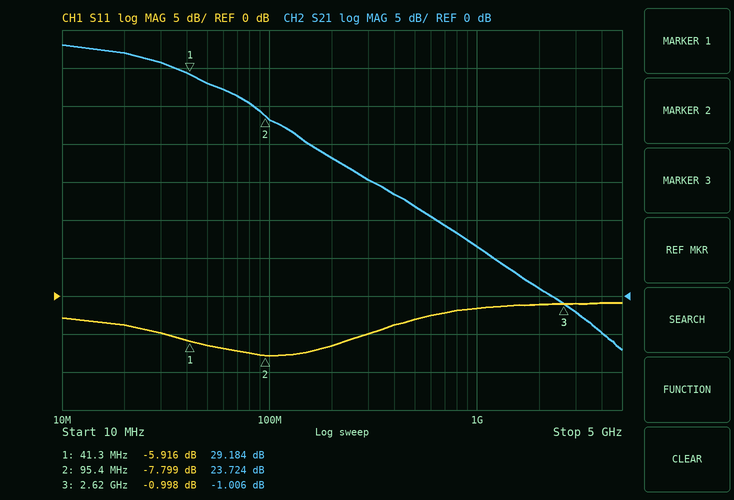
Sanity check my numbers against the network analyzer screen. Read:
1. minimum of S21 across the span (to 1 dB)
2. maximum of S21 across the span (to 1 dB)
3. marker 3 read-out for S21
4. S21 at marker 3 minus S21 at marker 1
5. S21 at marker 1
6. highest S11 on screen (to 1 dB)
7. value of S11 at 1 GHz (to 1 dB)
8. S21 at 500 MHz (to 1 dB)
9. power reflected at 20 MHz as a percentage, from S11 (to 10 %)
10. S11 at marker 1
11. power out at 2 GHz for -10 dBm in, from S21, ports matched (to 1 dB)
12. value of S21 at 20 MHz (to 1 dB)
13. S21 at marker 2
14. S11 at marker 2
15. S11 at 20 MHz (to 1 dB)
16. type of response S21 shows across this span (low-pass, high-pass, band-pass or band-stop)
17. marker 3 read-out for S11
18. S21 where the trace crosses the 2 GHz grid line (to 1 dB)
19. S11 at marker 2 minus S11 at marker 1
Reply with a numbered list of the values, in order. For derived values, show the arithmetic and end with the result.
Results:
1. -7 dB
2. 33 dB
3. -1.006 dB
4. -1.006 − (29.184) = -30.190 dB
5. 29.184 dB
6. -1 dB
7. -2 dB
8. 12 dB
9. 10^(-4/10) ≈ 40 %
10. -5.916 dB
11. -10 dBm + (1 dB) = -9 dBm
12. 32 dB
13. 23.724 dB
14. -7.799 dB
15. -4 dB
16. low-pass
17. -0.998 dB
18. 1 dB
19. -7.799 − (-5.916) = -1.883 dB
